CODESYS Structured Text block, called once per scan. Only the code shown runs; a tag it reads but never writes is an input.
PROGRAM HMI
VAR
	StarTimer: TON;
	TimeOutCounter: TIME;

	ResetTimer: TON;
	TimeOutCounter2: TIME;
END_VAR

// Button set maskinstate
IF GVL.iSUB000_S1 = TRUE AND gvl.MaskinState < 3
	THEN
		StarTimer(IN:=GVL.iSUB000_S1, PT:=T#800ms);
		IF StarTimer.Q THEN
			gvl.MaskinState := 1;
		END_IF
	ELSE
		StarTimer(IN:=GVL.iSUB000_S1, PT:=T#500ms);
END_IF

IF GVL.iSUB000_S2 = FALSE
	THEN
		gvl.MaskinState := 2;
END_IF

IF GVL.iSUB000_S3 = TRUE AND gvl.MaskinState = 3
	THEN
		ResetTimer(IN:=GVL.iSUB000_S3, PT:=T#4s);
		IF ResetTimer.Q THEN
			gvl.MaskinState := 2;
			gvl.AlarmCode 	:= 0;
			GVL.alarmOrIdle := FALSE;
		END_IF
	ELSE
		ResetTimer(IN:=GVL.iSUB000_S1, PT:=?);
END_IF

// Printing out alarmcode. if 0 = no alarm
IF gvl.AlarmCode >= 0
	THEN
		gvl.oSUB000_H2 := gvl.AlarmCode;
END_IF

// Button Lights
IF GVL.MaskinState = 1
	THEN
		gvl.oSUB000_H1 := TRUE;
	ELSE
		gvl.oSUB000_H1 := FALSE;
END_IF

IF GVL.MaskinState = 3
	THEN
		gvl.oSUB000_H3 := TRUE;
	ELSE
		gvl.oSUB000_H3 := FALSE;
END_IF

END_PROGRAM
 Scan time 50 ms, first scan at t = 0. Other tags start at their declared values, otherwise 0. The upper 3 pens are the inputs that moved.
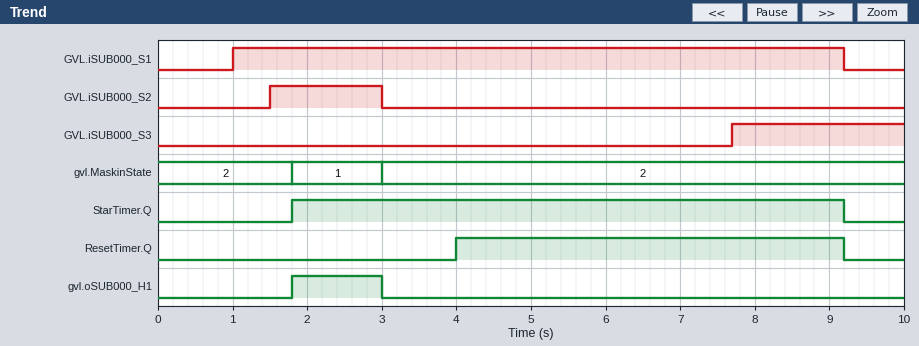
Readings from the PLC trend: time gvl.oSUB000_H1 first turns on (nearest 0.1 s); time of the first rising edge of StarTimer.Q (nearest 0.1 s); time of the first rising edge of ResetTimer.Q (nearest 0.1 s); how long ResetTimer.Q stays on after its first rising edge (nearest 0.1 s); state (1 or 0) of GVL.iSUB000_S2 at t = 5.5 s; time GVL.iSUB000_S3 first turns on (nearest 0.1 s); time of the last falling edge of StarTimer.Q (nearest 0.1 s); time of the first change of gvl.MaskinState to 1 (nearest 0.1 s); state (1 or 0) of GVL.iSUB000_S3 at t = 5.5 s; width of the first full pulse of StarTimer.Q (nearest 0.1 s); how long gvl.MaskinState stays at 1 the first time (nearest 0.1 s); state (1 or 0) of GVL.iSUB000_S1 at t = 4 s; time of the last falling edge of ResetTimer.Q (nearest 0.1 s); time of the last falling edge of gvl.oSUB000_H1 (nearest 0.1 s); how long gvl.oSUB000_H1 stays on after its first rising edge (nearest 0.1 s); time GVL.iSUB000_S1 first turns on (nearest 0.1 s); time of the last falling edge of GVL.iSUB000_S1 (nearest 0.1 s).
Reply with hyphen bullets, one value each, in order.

- 1.8 s
- 1.8 s
- 4.0 s
- 5.2 s
- 0
- 7.7 s
- 9.2 s
- 1.8 s
- 0
- 7.4 s
- 1.2 s
- 1
- 9.2 s
- 3.0 s
- 1.2 s
- 1.0 s
- 9.2 s
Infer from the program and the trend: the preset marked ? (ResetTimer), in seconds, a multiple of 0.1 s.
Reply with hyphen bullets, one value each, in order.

- 3.0 s
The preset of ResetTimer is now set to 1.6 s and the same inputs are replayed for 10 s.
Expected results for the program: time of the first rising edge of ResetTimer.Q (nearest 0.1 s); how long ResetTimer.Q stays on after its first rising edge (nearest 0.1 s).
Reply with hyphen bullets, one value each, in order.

- 2.6 s
- 6.6 s
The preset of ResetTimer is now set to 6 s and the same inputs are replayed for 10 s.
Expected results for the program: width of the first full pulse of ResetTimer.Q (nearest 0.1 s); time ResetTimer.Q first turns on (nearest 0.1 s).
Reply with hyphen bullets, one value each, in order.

- 2.2 s
- 7.0 s
